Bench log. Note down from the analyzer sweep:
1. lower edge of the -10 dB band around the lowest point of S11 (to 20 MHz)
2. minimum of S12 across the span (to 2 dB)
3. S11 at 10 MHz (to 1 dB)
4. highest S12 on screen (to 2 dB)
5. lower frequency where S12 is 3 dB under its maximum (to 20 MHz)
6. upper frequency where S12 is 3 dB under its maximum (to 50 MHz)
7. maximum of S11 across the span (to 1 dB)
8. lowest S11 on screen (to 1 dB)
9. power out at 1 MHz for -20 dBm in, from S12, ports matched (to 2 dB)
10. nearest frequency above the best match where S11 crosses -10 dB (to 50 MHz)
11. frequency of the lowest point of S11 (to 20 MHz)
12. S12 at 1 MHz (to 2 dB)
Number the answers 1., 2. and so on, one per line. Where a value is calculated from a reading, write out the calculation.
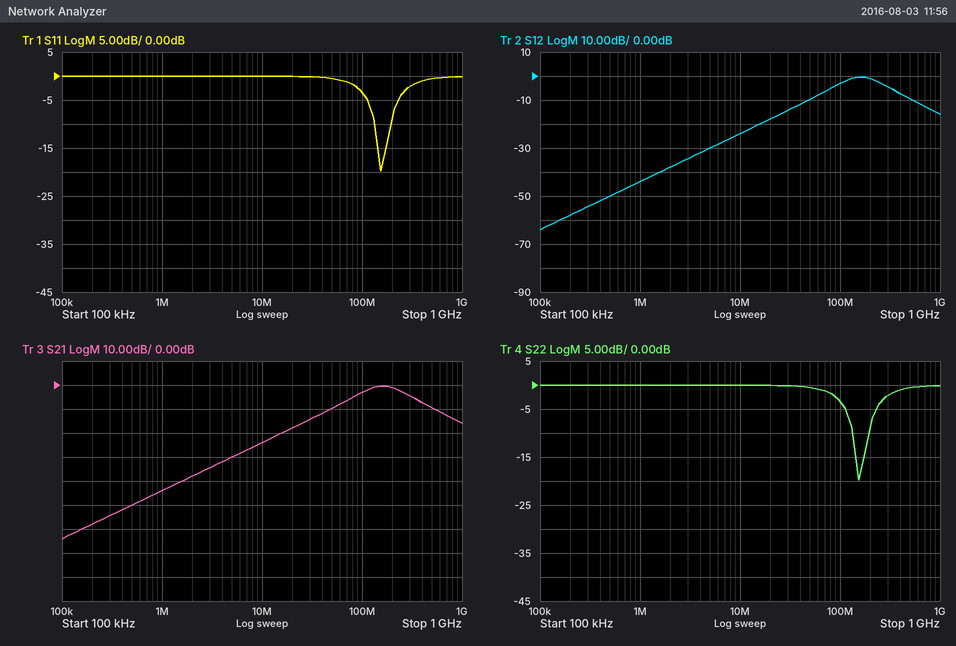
1. 140 MHz
2. -64 dB
3. 0 dB
4. 0 dB
5. 100 MHz
6. 250 MHz
7. 0 dB
8. -20 dB
9. -20 dBm + (-44 dB) = -64 dBm
10. 200 MHz
11. 160 MHz
12. -44 dB
